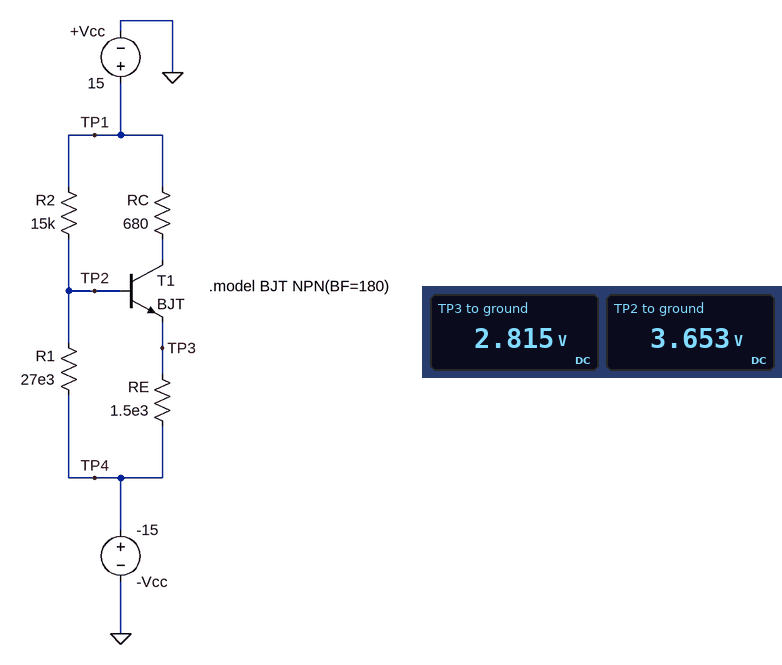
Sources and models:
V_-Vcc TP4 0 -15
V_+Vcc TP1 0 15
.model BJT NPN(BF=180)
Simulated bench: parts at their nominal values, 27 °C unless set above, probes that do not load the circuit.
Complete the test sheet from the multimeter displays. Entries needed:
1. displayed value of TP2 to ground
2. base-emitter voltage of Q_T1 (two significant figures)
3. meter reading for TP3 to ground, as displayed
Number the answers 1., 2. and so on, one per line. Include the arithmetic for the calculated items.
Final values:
1. 3.653 V
2. 3.653 V - 2.815 V = 840 mV
3. 2.815 V
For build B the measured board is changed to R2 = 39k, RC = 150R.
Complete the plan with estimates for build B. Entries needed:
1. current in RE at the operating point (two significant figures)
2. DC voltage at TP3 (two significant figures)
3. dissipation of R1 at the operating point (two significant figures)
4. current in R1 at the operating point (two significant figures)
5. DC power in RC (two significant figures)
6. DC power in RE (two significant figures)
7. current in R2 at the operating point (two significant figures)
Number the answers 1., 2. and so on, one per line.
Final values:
1. 7.2 mA
2. -4.2 V
3. 5.0 mW
4. 430 µA
5. 7.7 mW
6. 78 mW
7. 470 µA
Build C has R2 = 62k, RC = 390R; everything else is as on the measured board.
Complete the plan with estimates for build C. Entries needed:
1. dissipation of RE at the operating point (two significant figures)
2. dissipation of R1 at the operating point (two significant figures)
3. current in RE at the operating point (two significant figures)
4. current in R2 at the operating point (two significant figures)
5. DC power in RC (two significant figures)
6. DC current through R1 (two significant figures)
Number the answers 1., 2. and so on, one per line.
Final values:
1. 40 mW
2. 2.7 mW
3. 5.2 mA
4. 350 µA
5. 10 mW
6. 320 µA
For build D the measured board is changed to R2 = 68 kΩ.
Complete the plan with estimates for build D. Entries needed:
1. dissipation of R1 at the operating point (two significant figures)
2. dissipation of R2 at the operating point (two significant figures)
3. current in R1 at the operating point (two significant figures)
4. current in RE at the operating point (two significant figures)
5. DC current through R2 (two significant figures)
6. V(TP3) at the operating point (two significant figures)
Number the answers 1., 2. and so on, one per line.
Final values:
1. 2.4 mW
2. 7.1 mW
3. 300 µA
4. 4.8 mA
5. 320 µA
6. -7.8 V
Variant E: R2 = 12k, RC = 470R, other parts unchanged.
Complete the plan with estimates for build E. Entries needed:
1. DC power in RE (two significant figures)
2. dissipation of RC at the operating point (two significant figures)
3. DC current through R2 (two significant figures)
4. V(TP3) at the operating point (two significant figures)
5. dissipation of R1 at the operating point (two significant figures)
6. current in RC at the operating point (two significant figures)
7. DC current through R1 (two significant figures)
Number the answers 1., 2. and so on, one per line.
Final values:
1. 250 mW
2. 77 mW
3. 820 µA
4. 4.3 V
5. 15 mW
6. 13 mA
7. 750 µA
